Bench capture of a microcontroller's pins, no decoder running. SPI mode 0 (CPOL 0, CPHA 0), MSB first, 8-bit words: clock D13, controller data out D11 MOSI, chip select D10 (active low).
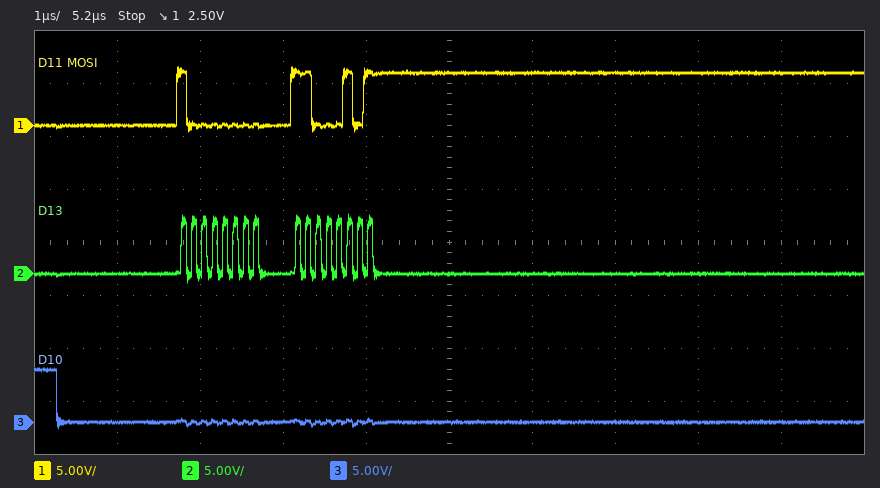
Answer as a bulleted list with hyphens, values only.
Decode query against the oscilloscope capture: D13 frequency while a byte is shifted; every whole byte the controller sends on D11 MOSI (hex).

- 8 MHz
- 80 C5
